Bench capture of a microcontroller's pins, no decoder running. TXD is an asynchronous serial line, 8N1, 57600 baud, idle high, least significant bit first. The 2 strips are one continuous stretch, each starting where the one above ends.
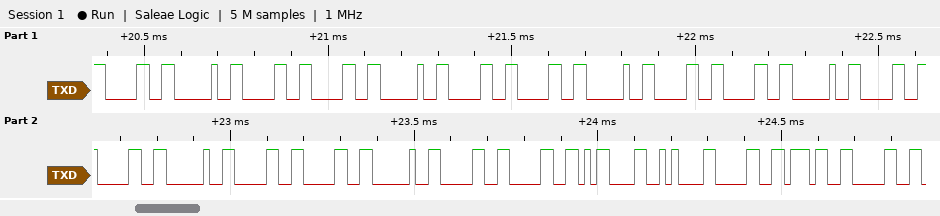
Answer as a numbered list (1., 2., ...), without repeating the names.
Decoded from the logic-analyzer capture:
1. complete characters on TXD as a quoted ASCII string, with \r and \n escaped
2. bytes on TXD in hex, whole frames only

1. "0 00 00 00 00 00 00\r\n070"
2. 30 20 30 30 20 30 30 20 30 30 20 30 30 20 30 30 20 30 30 0D 0A 30 37 30
